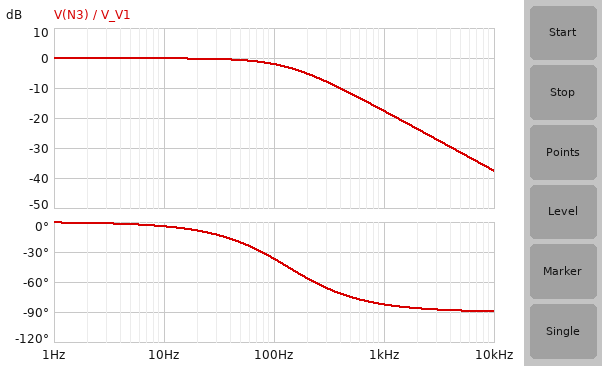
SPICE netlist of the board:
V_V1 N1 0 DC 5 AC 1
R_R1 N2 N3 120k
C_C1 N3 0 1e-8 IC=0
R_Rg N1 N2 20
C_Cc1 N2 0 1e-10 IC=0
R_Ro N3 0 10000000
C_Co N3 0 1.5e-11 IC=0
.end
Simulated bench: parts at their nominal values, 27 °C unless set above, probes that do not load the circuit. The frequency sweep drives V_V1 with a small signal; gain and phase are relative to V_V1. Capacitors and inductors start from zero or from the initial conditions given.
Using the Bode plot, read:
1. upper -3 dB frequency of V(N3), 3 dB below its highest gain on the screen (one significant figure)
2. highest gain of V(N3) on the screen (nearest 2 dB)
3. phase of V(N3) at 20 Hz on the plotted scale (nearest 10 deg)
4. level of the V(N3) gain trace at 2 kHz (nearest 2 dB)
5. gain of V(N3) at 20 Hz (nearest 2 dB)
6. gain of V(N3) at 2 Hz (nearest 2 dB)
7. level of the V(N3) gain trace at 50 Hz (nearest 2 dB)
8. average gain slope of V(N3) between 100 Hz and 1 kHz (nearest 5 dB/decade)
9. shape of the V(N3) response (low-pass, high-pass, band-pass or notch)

100 Hz
0 dB
-10 deg
-24 dB
0 dB
0 dB
0 dB
-15 dB/decade
low-pass
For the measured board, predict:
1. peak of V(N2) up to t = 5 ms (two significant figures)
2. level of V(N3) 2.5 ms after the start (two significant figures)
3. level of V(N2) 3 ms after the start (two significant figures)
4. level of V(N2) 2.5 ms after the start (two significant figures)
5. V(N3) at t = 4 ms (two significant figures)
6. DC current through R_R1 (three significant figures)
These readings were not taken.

5.0 V
4.3 V
5.0 V
5.0 V
4.8 V
494 nA
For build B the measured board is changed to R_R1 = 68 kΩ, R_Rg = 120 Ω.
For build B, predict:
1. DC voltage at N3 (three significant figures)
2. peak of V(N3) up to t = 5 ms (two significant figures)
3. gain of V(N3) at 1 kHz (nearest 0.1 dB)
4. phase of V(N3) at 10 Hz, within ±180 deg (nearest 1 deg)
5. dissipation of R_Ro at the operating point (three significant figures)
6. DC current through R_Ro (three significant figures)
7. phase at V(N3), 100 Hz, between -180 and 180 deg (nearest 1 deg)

4.97 V
5.0 V
-12.9 dB
-2 deg
2.47 µW
497 nA
-23 deg
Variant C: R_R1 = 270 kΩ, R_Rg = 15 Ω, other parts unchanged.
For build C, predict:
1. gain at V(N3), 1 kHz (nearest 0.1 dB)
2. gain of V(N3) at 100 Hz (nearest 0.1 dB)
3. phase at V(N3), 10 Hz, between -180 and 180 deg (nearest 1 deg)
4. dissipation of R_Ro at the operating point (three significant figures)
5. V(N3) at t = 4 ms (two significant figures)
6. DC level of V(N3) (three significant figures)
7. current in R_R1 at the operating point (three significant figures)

-24.6 dB
-6.0 dB
-9 deg
2.37 µW
3.8 V
4.87 V
487 nA
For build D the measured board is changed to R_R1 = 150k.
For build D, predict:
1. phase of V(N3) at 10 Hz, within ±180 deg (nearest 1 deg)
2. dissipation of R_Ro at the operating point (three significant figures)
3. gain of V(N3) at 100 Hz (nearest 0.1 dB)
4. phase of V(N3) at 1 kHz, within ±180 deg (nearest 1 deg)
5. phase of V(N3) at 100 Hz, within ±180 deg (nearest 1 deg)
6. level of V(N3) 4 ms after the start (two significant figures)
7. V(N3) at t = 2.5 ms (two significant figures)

-5 deg
2.43 µW
-2.8 dB
-84 deg
-43 deg
4.6 V
4.0 V
